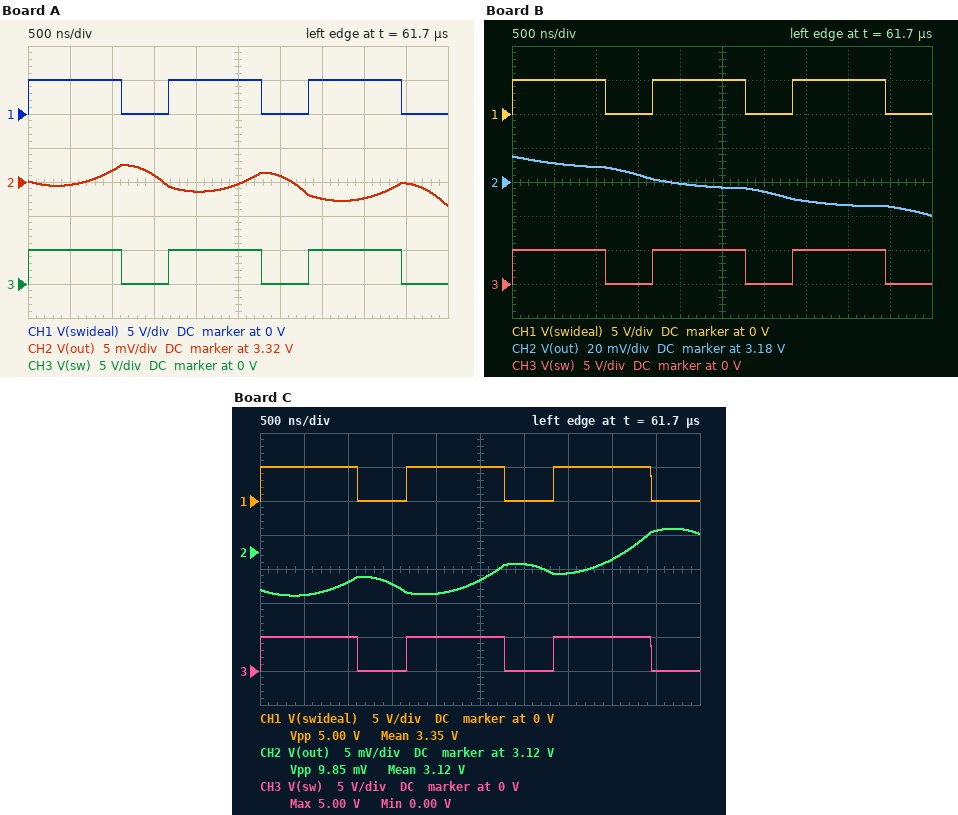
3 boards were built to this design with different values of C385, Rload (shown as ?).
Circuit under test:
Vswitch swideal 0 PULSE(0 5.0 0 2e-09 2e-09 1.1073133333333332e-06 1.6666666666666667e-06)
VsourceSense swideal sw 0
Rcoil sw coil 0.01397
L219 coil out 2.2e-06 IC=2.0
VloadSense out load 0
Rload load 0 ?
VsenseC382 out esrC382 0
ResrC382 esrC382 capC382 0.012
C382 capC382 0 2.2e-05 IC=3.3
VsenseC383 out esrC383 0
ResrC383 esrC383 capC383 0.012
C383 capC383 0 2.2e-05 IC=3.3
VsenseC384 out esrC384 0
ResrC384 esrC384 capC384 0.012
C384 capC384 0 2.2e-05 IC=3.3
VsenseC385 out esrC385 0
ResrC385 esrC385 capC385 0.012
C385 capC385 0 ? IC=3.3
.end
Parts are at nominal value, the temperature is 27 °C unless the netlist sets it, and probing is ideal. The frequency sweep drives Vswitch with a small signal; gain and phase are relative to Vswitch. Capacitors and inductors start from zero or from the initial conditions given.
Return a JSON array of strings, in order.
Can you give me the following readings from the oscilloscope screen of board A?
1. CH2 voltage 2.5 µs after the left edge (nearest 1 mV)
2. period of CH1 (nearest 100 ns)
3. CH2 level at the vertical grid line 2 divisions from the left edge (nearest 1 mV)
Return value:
["3.320 V", "1.7 µs", "3.322 V"]
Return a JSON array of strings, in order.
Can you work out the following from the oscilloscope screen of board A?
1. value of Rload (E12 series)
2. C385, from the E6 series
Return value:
["1.2 Ω", "6.8 µF"]
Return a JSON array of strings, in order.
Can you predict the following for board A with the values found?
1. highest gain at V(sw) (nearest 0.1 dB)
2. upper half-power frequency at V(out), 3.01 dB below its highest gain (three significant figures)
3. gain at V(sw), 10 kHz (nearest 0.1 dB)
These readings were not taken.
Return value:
["0 dB", "13.9 kHz", "0 dB"]
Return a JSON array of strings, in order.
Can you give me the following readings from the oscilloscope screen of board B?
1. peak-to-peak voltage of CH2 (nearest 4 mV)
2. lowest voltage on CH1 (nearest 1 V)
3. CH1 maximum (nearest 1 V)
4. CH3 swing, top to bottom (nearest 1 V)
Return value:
["36 mV", "0 V", "5 V", "5 V"]
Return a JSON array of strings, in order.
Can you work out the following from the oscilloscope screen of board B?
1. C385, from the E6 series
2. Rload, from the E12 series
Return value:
["47 µF", "5.6 Ω"]
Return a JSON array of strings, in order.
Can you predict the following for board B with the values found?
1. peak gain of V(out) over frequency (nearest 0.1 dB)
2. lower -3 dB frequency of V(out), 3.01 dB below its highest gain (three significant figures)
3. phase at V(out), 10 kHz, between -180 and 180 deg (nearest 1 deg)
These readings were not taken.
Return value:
["16.5 dB", "9.26 kHz", "-81 deg"]
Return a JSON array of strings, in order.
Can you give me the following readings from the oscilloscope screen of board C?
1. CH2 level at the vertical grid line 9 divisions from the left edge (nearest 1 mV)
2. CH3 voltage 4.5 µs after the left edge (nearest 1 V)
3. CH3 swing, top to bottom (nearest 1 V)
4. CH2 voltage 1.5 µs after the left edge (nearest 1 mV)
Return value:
["3.123 V", "0 V", "5 V", "3.115 V"]
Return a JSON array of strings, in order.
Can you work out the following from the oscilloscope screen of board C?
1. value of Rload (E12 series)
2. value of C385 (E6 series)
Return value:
["4.7 Ω", "15 µF"]
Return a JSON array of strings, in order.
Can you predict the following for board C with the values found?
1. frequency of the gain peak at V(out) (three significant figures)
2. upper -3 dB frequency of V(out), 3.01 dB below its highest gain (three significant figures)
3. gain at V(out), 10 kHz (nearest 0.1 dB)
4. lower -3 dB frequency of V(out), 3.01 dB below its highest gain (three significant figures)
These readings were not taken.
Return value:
["11.9 kHz", "12.7 kHz", "9.9 dB", "11.0 kHz"]
